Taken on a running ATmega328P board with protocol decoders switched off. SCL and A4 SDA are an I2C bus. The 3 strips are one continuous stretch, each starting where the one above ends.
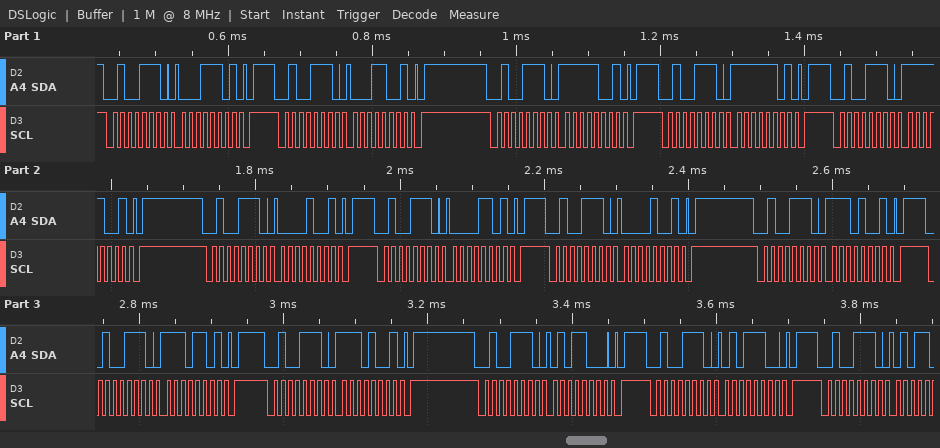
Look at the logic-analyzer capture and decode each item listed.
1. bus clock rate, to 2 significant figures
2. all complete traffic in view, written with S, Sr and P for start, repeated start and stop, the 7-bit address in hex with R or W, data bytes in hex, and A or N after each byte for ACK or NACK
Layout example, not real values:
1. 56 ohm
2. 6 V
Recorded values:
1. 100 kHz
2. S 27W A 1D A P S 27W A 19 A P S 27W A F9 A P S 27W A FD A P S 27W A F9 A P S 27W A 09 A P S 27W A 0D A P S 27W A 09 A P S 27W A E9 A P S 27W A ED A P S 27W A E9 A P S 27W A 58 A P S 27W A 5C A P S 27W A
